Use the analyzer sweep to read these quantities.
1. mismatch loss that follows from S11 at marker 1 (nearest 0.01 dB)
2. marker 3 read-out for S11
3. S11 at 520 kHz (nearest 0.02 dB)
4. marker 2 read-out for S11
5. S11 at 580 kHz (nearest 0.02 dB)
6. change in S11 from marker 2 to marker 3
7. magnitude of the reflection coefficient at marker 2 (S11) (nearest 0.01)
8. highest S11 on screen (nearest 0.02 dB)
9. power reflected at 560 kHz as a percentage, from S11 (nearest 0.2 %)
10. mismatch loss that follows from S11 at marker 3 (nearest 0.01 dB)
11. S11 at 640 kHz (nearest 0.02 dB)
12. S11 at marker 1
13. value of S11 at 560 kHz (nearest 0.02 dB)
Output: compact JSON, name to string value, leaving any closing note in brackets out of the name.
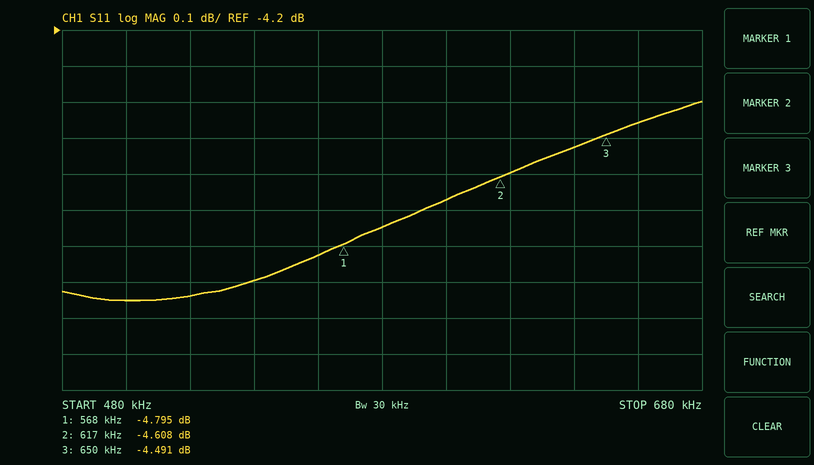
{"mismatch loss that follows from S11 at marker 1": "1.75 dB", "marker 3 read-out for S11": "-4.491 dB", "S11 at 520 kHz": "-4.94 dB", "marker 2 read-out for S11": "-4.608 dB", "S11 at 580 kHz": "-4.74 dB", "change in S11 from marker 2 to marker 3": "0.117 dB", "magnitude of the reflection coefficient at marker 2 (S11)": "0.59", "highest S11 on screen": "-4.40 dB", "power reflected at 560 kHz as a percentage, from S11": "33.0 %", "mismatch loss that follows from S11 at marker 3": "1.91 dB", "S11 at 640 kHz": "-4.52 dB", "S11 at marker 1": "-4.795 dB", "value of S11 at 560 kHz": "-4.82 dB"}
